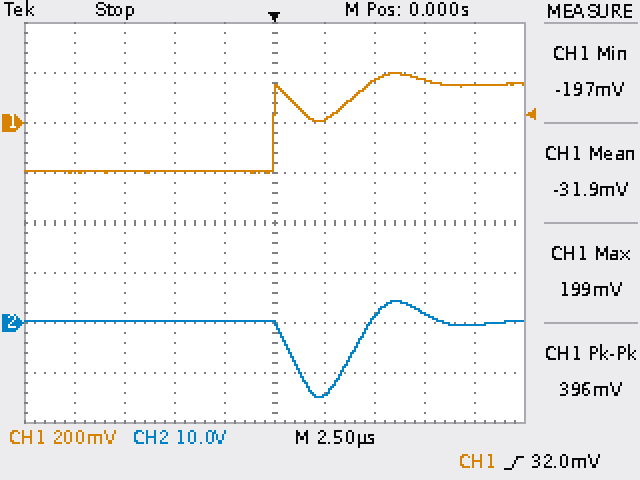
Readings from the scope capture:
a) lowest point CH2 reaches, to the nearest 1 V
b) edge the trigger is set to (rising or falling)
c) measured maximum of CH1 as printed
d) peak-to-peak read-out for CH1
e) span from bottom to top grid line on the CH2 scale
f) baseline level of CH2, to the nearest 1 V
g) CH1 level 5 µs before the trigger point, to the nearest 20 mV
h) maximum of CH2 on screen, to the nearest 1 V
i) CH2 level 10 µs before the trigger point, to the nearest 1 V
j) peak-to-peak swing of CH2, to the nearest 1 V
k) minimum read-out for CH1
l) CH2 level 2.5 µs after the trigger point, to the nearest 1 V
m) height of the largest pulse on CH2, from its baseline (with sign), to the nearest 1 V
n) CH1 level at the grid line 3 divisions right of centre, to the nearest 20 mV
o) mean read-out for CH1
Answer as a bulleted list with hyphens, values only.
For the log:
- -15 V
- rising
- 199 mV
- 396 mV
- 80 V
- 0 V
- -200 mV
- 4 V
- 0 V
- 19 V
- -197 mV
- -14 V
- -15 V
- 180 mV
- -31.9 mV
